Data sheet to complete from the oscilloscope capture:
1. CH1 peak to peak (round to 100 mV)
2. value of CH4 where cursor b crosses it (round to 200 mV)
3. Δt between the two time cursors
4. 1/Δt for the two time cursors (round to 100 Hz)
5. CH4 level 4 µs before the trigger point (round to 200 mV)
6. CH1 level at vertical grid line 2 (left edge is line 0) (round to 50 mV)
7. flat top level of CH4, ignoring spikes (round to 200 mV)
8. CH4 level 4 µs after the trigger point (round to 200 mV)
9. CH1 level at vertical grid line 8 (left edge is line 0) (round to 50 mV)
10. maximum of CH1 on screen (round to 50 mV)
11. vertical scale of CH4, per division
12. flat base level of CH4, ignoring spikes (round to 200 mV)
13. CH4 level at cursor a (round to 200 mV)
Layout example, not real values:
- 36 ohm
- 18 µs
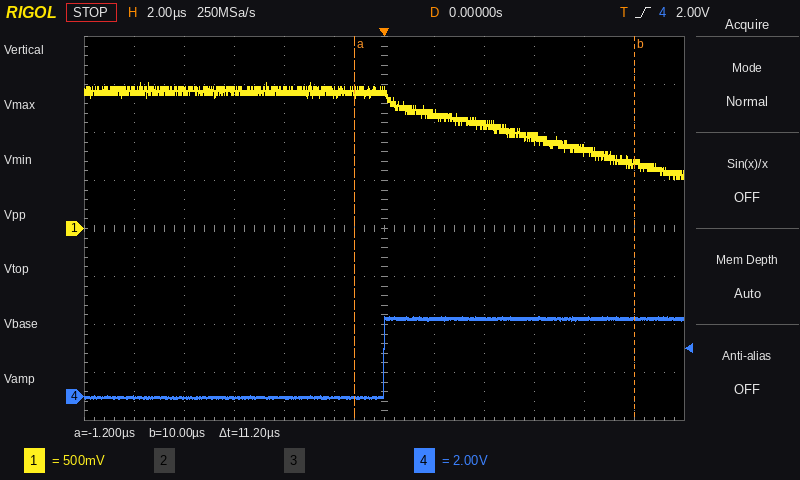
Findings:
- 1.00 V
- 3.2 V
- 11.2 µs
- 89.3 kHz
- 0.0 V
- 1.45 V
- 3.2 V
- 3.2 V
- 1.10 V
- 1.50 V
- 2 V
- 0.0 V
- 0.0 V
